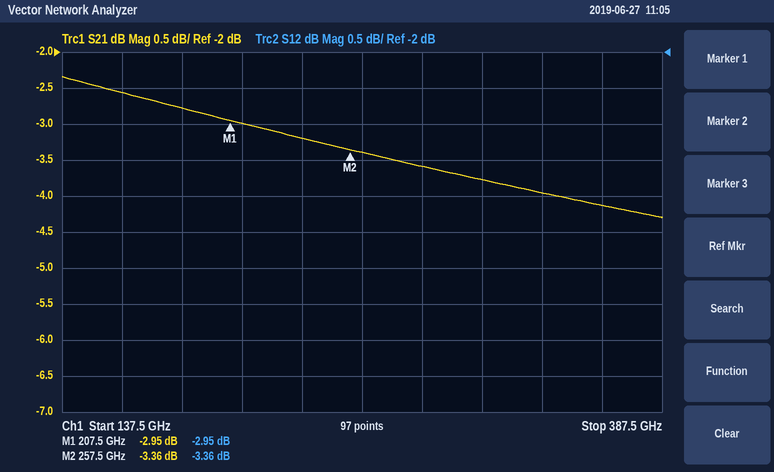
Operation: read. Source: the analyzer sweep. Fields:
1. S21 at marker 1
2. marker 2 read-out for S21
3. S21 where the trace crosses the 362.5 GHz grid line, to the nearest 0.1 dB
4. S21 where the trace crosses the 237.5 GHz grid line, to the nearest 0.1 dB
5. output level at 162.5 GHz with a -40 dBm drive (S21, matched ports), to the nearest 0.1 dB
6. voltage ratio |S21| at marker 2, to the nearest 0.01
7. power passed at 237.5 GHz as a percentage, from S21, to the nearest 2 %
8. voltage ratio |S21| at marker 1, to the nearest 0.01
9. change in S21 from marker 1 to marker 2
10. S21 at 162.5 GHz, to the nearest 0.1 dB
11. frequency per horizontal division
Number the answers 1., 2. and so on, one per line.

1. -2.95 dB
2. -3.36 dB
3. -4.1 dB
4. -3.2 dB
5. -42.6 dBm
6. 0.68
7. 48 %
8. 0.71
9. -0.41 dB
10. -2.6 dB
11. 25 GHz
